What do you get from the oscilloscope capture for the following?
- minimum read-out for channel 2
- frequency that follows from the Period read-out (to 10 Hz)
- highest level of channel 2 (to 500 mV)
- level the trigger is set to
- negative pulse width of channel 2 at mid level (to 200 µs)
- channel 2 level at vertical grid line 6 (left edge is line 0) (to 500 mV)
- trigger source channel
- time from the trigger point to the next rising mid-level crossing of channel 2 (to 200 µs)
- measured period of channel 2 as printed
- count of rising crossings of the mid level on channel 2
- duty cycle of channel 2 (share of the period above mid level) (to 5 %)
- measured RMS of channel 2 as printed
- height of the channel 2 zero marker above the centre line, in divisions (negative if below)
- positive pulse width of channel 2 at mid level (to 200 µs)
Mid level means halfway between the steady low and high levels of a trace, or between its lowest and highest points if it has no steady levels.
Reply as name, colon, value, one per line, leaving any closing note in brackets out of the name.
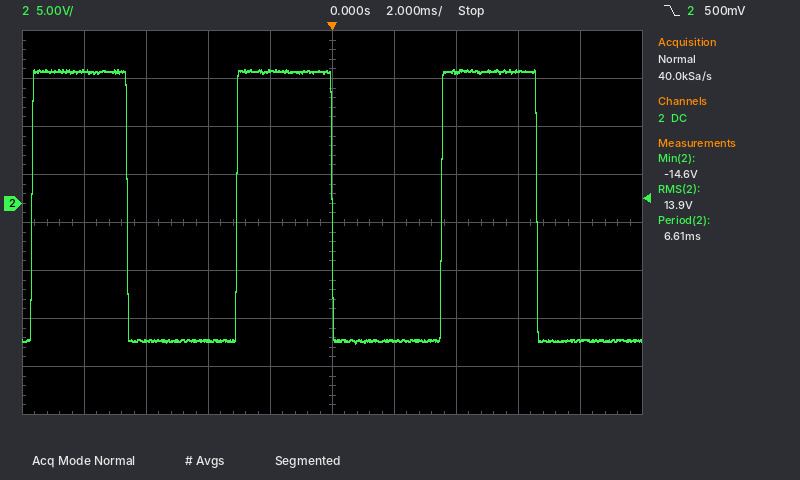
minimum read-out for channel 2: -14.6 V
frequency that follows from the Period read-out: 150 Hz
highest level of channel 2: 14.0 V
level the trigger is set to: 500 mV
negative pulse width of channel 2 at mid level: 3.6 ms
channel 2 level at vertical grid line 6 (left edge is line 0): -14.5 V
trigger source channel: channel 2
time from the trigger point to the next rising mid-level crossing of channel 2: 3.6 ms
measured period of channel 2 as printed: 6.61 ms
count of rising crossings of the mid level on channel 2: 3
duty cycle of channel 2 (share of the period above mid level): 45 %
measured RMS of channel 2 as printed: 13.9 V
height of the channel 2 zero marker above the centre line, in divisions: +0.4 div
positive pulse width of channel 2 at mid level: 3.0 ms
